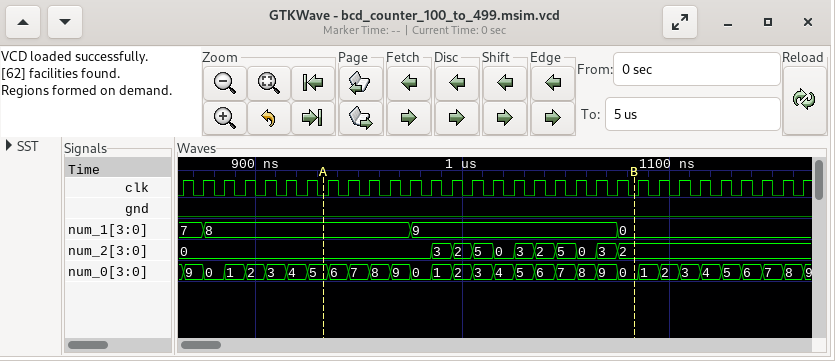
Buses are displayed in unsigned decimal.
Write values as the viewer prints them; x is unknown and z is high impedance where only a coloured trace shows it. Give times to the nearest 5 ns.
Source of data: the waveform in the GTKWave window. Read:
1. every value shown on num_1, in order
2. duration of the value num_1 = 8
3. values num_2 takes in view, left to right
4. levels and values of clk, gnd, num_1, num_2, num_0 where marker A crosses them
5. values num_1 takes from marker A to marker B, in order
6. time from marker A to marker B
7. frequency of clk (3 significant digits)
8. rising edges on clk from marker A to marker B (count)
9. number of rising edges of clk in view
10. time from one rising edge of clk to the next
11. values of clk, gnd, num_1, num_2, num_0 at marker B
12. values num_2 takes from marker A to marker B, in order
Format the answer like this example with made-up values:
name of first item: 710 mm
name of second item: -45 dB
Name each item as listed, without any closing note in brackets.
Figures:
every value shown on num_1, in order: 7, 8, 9, 0
duration of the value num_1 = 8: 100 ns
values num_2 takes in view, left to right: 0, 3, 2, 5, 0, 3, 2, 5, 0, 3, 2
levels and values of clk, gnd, num_1, num_2, num_0 where marker A crosses them: clk=0, gnd=0, num_1=8, num_2=0, num_0=5
values num_1 takes from marker A to marker B, in order: 8, 9, 0
time from marker A to marker B: 150 ns
frequency of clk: 100 MHz
rising edges on clk from marker A to marker B: 15
number of rising edges of clk in view: 31
time from one rising edge of clk to the next: 10 ns
values of clk, gnd, num_1, num_2, num_0 at marker B: clk=0, gnd=0, num_1=0, num_2=2, num_0=0
values num_2 takes from marker A to marker B, in order: 0, 3, 2, 5, 0, 3, 2, 5, 0, 3, 2
